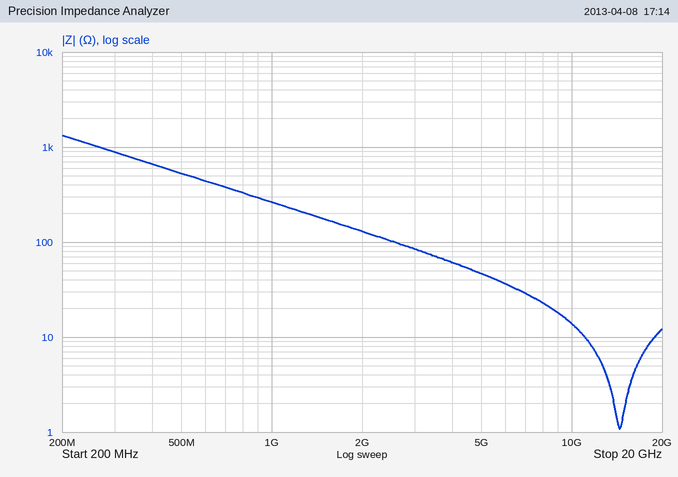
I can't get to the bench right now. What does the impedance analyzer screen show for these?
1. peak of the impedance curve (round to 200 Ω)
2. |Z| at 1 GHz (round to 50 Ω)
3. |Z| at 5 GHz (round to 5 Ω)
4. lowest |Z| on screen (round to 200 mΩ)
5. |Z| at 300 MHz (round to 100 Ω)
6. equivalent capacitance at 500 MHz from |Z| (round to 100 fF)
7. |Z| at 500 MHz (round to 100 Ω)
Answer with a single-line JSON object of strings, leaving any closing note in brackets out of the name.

{"peak of the impedance curve": "1.4 kΩ", "|Z| at 1 GHz": "250 Ω", "|Z| at 5 GHz": "45 Ω", "lowest |Z| on screen": "1.0 Ω", "|Z| at 300 MHz": "900 Ω", "equivalent capacitance at 500 MHz from |Z|": "600 fF", "|Z| at 500 MHz": "500 Ω"}
